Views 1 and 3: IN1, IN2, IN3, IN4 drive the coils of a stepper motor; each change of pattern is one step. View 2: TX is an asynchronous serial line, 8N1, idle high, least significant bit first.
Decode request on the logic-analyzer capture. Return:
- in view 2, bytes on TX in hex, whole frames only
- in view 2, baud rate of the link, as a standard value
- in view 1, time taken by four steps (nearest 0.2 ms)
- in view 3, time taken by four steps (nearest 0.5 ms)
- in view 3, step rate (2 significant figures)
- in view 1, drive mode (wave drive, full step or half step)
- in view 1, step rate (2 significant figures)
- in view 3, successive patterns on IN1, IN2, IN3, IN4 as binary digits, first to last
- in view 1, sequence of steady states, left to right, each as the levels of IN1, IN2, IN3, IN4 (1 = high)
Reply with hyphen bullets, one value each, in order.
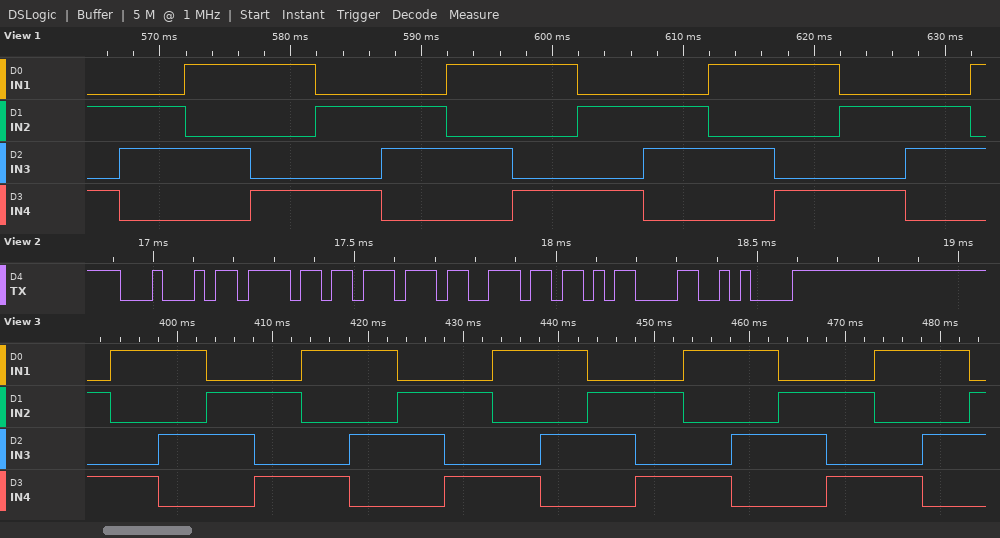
- 44 6F 77 6E 0D 0A
- 38400 baud
- 20.0 ms
- 20.0 ms
- 200 steps/s
- full step
- 200 steps/s
- 0101 1001 1010 0110 0101 1001 1010 0110 0101 1001 1010 0110 0101 1001 1010 0110 0101 1001 1010 0110
- 0101 0110 1010 1001 0101 0110 1010 1001 0101 0110 1010 1001 0101 0110 1010
